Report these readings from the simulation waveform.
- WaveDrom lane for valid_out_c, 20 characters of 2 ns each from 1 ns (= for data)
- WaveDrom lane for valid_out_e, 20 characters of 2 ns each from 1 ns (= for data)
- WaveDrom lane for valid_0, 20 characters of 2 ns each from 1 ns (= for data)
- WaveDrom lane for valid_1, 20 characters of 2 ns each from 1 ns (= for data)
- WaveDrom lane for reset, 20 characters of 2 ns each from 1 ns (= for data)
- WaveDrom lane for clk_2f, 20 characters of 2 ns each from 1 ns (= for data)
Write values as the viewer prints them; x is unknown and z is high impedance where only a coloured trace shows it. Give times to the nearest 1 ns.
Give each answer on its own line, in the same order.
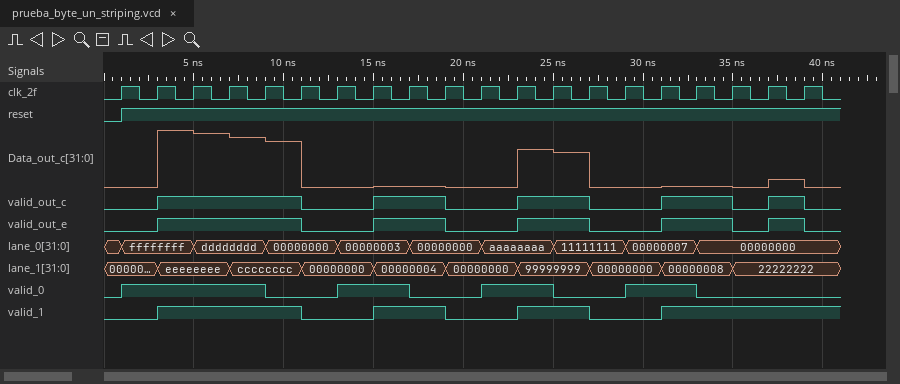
{name: 'valid_out_c', wave: '01...0.1.0.1.0.1.010'}
{name: 'valid_out_e', wave: '01...0.1.0.1.0.1.010'}
{name: 'valid_0', wave: '1...0.1.0.1.0.1.0...'}
{name: 'valid_1', wave: '01...0.1.0.1.0.1....'}
{name: 'reset', wave: '1...................'}
{name: 'clk_2f', wave: 'p...................'}
